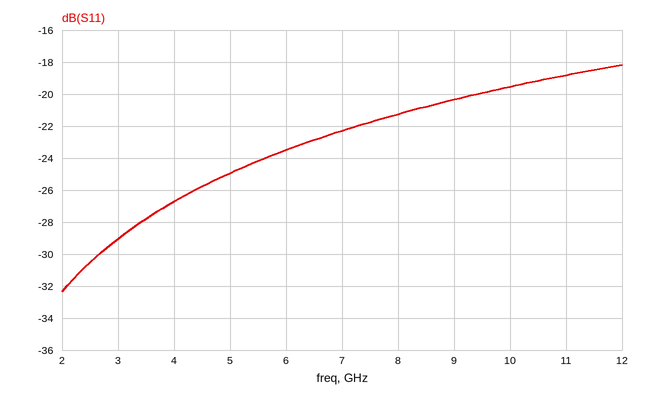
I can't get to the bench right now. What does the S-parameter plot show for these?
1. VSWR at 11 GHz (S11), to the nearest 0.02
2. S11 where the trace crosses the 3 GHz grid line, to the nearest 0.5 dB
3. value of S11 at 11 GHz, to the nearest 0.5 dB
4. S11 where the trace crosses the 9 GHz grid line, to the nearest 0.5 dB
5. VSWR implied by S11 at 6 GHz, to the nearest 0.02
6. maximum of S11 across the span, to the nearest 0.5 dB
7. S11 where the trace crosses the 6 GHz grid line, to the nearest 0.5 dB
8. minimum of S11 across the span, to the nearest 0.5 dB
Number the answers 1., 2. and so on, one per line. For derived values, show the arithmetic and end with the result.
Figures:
1. |Γ| = 10^(-19/20) = 0.1122; VSWR = (1 + 0.1122)/(1 − 0.1122) ≈ 1.25, so 1.26 to the nearest 0.02
2. -29.0 dB
3. -19.0 dB
4. -20.5 dB
5. |Γ| = 10^(-23.5/20) = 0.0668; VSWR = (1 + 0.0668)/(1 − 0.0668) ≈ 1.14
6. -18.0 dB
7. -23.5 dB
8. -32.5 dB
